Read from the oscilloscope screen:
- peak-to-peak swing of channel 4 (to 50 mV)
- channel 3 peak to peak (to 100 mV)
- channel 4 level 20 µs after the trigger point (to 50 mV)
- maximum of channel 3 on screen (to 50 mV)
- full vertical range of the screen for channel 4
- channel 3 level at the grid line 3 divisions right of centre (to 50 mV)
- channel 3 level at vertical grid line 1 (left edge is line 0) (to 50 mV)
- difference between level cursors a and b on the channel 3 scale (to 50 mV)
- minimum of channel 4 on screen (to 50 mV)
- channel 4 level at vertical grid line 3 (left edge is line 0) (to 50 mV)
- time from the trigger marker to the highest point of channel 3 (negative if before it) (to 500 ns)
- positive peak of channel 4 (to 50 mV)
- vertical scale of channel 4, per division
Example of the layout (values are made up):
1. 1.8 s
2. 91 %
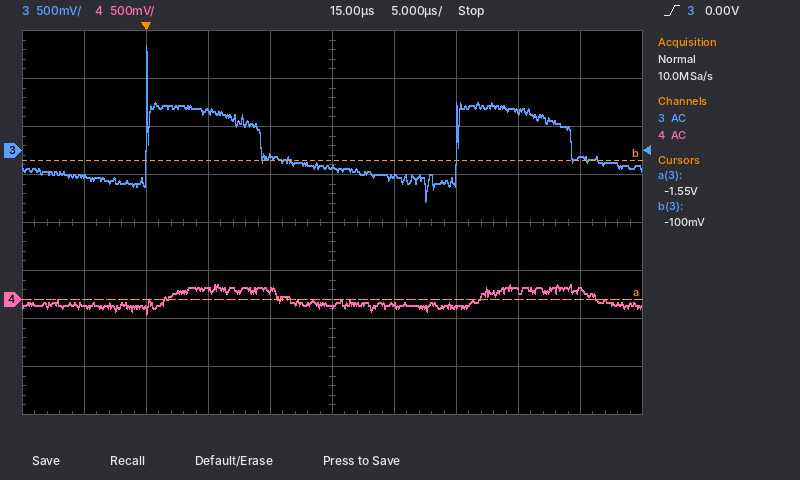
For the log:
1. 300 mV
2. 1.60 V
3. -50 mV
4. 1.10 V
5. 4 V
6. 400 mV
7. -250 mV
8. 1.45 V
9. -150 mV
10. 100 mV
11. 0.0 µs
12. 150 mV
13. 500 mV
